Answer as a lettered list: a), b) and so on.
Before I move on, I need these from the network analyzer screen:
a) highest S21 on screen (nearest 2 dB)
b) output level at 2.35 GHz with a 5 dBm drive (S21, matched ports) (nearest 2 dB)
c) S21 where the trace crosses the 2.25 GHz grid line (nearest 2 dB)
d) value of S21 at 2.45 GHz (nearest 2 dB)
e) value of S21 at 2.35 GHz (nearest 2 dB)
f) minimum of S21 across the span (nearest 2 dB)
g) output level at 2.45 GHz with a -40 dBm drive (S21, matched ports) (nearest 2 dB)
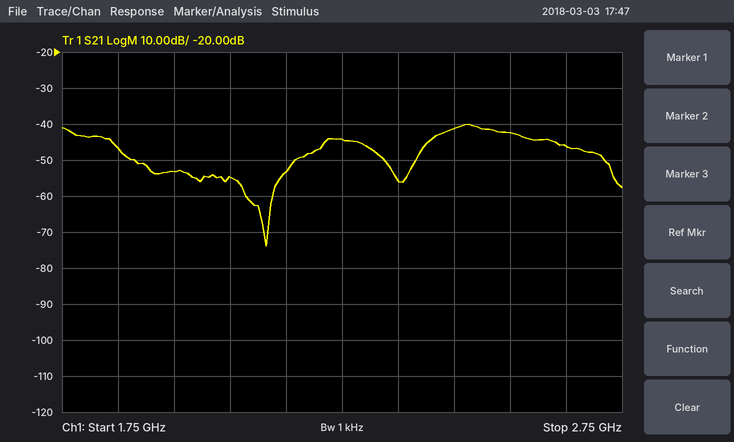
a) -40 dB
b) -50 dBm
c) -44 dB
d) -42 dB
e) -56 dB
f) -74 dB
g) -82 dBm
